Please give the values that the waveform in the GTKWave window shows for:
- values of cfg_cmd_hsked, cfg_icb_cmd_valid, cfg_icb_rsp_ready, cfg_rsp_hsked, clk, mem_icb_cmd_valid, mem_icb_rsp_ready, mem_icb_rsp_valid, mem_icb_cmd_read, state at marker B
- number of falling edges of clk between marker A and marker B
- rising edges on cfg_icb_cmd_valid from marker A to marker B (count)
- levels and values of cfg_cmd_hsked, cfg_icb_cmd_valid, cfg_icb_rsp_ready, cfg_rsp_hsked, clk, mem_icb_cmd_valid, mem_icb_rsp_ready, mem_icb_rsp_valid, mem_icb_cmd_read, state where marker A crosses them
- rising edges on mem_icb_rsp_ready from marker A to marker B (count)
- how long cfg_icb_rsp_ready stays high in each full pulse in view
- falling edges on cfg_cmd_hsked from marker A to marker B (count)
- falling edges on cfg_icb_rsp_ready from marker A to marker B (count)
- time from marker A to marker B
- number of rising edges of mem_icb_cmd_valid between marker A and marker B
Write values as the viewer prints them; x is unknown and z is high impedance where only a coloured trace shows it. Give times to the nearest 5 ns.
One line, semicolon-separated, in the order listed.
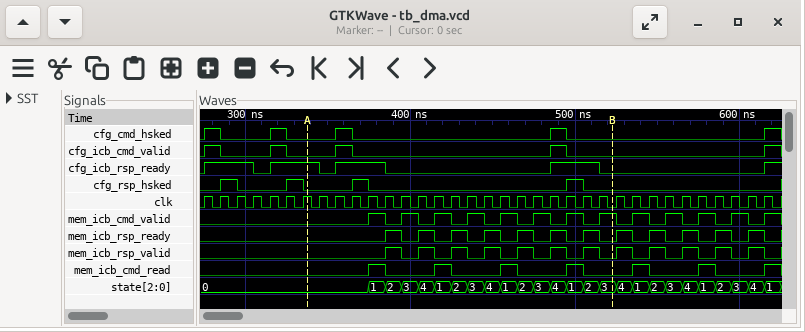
cfg_cmd_hsked=0, cfg_icb_cmd_valid=0, cfg_icb_rsp_ready=0, cfg_rsp_hsked=0, clk=0, mem_icb_cmd_valid=1, mem_icb_rsp_ready=0, mem_icb_rsp_valid=0, mem_icb_cmd_read=0, state=3; 19; 2; cfg_cmd_hsked=0, cfg_icb_cmd_valid=0, cfg_icb_rsp_ready=1, cfg_rsp_hsked=0, clk=1, mem_icb_cmd_valid=0, mem_icb_rsp_ready=0, mem_icb_rsp_valid=0, mem_icb_cmd_read=0, state=0; 7; 30 ns, 30 ns, 30 ns, 30 ns; 2; 3; 185 ns; 8
